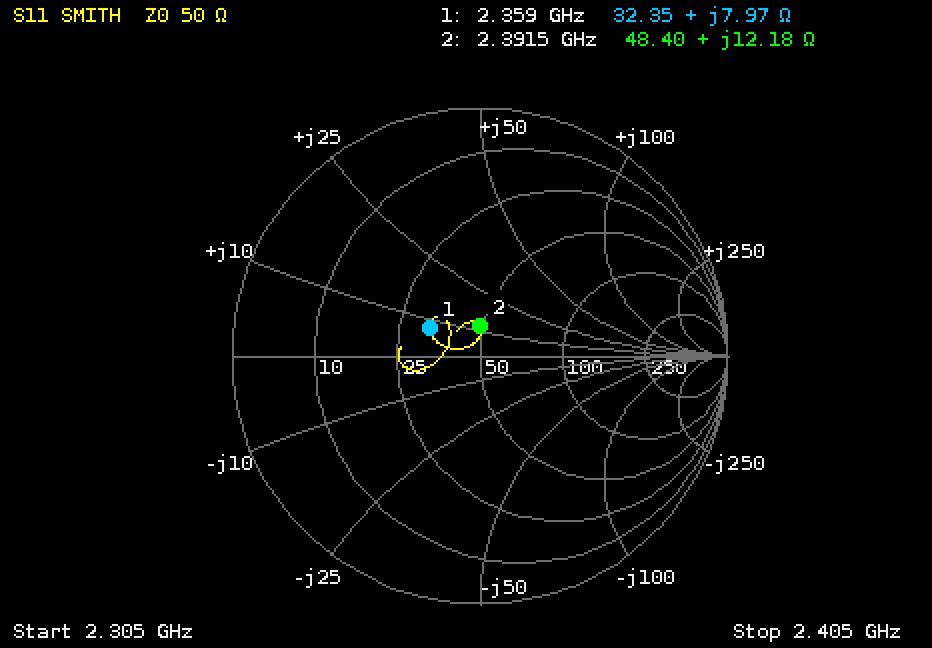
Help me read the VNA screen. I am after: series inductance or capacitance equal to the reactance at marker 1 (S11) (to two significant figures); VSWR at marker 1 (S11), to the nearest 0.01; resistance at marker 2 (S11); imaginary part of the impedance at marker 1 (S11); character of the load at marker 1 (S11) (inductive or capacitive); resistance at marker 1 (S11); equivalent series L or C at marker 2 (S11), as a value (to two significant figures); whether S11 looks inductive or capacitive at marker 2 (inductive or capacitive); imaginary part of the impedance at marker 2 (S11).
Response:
540 pH
1.61
48.40 Ω
+7.97 Ω
inductive
32.35 Ω
810 pH
inductive
+12.18 Ω
